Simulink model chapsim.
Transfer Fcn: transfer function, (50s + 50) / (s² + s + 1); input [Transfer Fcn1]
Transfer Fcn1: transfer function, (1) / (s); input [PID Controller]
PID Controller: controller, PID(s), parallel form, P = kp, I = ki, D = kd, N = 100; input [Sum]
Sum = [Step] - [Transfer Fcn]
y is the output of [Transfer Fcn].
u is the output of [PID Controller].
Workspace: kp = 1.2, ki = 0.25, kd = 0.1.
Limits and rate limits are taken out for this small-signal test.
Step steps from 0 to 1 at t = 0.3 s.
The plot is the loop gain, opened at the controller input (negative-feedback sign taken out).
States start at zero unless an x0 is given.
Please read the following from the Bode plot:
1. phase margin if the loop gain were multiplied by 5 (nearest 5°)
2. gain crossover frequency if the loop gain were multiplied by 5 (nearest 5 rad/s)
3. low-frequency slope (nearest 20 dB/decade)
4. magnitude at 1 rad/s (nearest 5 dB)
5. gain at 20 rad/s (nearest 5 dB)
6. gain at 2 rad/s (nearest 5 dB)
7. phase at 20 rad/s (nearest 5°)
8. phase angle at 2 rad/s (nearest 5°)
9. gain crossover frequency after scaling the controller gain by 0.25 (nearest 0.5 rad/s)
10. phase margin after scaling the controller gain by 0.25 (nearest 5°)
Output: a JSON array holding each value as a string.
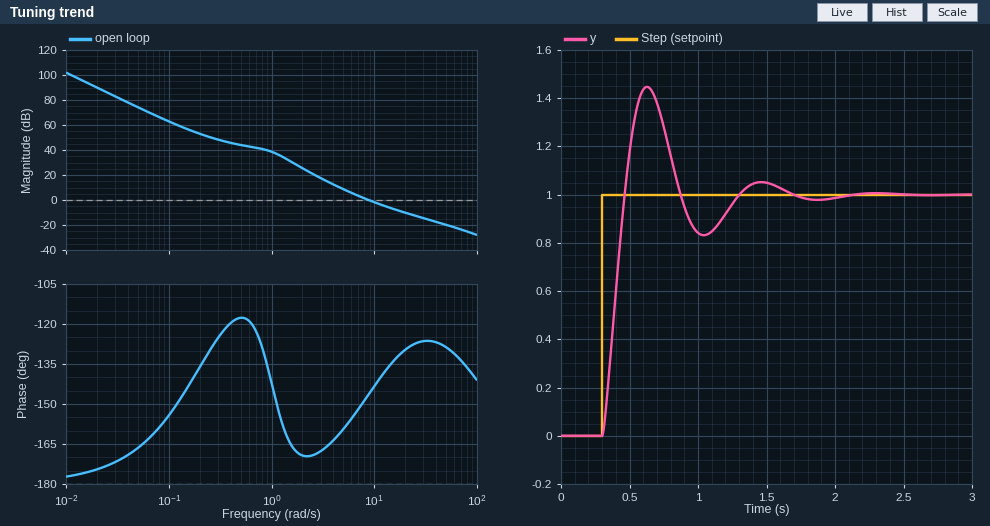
["55°", "30 rad/s", "-40 dB/decade", "40 dB", "-10 dB", "25 dB", "-130°", "-170°", "4.0 rad/s", "15°"]
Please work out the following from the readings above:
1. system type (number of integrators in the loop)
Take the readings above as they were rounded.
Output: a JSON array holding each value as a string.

["2"]
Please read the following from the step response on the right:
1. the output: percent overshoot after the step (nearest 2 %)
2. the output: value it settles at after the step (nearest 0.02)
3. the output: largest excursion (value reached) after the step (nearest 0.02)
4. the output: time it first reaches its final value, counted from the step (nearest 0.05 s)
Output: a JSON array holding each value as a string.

["44 %", "1.00", "1.44", "0.15 s"]
